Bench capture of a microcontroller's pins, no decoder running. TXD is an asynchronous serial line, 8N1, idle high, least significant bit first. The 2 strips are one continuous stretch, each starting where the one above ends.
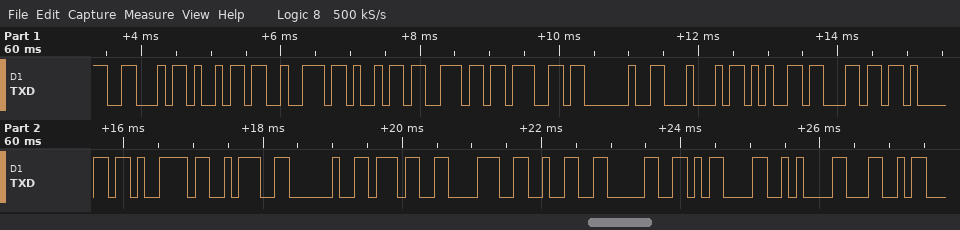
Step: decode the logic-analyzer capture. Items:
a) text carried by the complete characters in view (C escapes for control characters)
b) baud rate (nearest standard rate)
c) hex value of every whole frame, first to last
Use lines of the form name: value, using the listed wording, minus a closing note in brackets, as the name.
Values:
text carried by the complete characters in view: "Firing Delay: 7820\r\nL"
baud rate: 9600 baud
hex value of every whole frame, first to last: 46 69 72 69 6E 67 20 44 65 6C 61 79 3A 20 37 38 32 30 0D 0A 4C
